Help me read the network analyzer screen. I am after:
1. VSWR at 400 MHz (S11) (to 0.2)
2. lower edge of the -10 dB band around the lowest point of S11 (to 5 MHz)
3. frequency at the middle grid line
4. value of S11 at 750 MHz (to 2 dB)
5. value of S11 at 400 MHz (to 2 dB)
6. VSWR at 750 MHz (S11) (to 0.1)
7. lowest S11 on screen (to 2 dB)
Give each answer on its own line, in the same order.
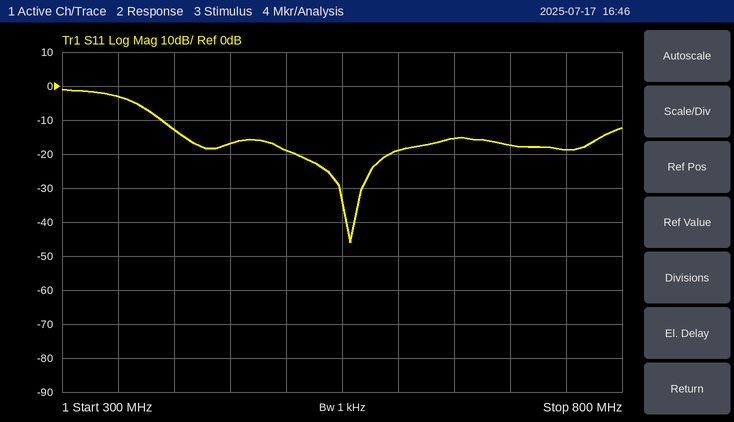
1.6
390 MHz
550 MHz
-18 dB
-12 dB
1.3
-46 dB
